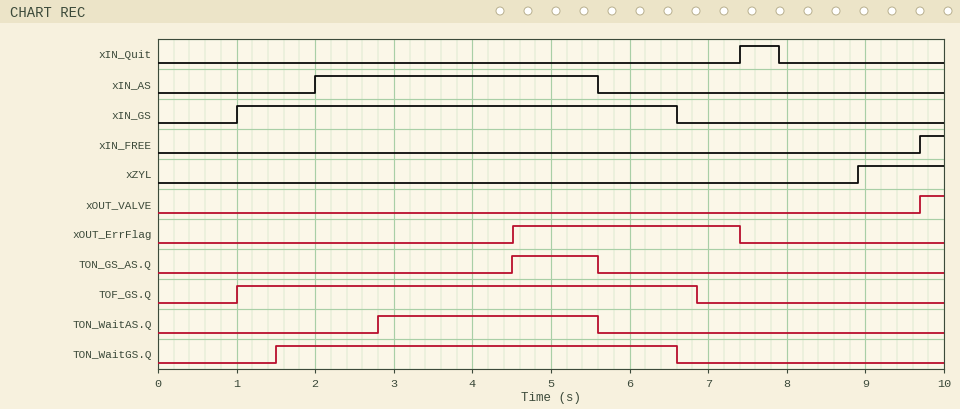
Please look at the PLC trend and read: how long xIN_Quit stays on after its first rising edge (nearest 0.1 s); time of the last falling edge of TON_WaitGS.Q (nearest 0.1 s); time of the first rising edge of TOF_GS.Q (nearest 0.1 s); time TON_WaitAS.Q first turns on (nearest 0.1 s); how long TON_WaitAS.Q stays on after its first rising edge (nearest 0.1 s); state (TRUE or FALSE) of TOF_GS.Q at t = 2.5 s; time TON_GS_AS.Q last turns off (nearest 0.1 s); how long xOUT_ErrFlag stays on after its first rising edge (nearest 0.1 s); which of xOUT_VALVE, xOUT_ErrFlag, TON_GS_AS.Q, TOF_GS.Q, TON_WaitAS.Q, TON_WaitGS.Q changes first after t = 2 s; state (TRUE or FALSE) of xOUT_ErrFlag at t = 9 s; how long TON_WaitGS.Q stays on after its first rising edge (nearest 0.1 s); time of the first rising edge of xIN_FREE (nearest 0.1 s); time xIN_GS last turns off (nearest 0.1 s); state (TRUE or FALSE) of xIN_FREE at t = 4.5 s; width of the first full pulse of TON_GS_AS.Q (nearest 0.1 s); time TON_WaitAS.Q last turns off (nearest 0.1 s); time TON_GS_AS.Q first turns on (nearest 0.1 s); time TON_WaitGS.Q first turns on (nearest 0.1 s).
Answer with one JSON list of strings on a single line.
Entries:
["0.5 s", "6.6 s", "1.0 s", "2.8 s", "2.8 s", "TRUE", "5.6 s", "2.9 s", "TON_WaitAS.Q", "FALSE", "5.1 s", "9.7 s", "6.6 s", "FALSE", "1.1 s", "5.6 s", "4.5 s", "1.5 s"]
